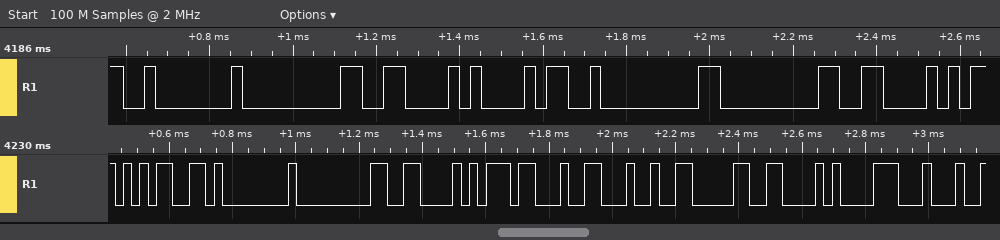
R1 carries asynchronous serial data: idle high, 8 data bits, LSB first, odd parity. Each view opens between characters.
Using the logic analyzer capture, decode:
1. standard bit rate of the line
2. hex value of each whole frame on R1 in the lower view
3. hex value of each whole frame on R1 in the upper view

38400 baud
35, 01, 00, 86, 37, 46, 06, 86, 38
02, 00, 86, 68, 00, 00, 86
